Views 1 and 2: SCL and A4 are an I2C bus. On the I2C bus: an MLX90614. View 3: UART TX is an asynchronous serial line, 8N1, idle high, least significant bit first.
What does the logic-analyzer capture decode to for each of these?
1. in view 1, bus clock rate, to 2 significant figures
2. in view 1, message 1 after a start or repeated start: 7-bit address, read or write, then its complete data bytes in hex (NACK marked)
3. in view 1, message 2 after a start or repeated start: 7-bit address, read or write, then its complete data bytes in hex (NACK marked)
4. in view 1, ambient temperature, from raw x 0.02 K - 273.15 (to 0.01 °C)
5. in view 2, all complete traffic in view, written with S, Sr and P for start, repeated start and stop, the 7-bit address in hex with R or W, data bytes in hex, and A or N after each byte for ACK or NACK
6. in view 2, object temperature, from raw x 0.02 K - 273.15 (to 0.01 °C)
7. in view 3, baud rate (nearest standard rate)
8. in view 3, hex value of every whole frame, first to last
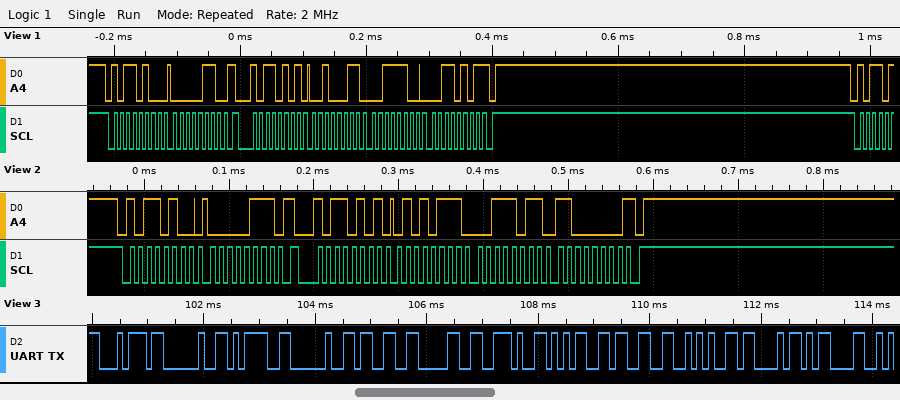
100 kHz
0x5A write: 06
0x5A read: 23 3C 35 NACK
34.75 °C
S 5AW A 07 A Sr 5AR A 57 A 3B A C0 N P
30.67 °C
9600 baud
0x74 0x20 0x3D 0x20 0x33 0x30 0x2E 0x35 0x33 0x2A 0x43 0x0D
